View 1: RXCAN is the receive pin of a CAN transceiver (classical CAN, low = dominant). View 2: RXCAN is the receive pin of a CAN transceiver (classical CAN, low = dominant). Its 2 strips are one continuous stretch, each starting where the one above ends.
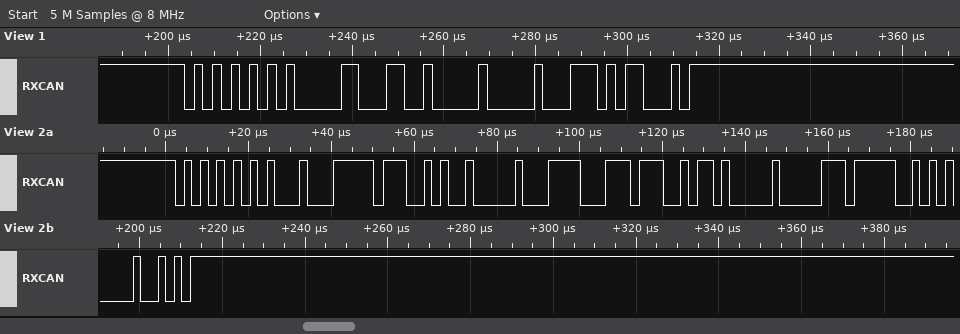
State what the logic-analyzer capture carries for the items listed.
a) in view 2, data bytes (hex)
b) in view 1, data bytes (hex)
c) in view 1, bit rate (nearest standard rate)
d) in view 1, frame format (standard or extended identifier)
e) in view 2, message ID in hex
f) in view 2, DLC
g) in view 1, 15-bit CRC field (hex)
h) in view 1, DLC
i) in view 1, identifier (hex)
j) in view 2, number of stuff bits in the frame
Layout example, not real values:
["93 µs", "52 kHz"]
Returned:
["FF 29 00 F1 DC B4 00 DF", "32 00", "500 kbit/s", "standard", "0x555", "8", "0x0758", "2", "0x555", "5"]
